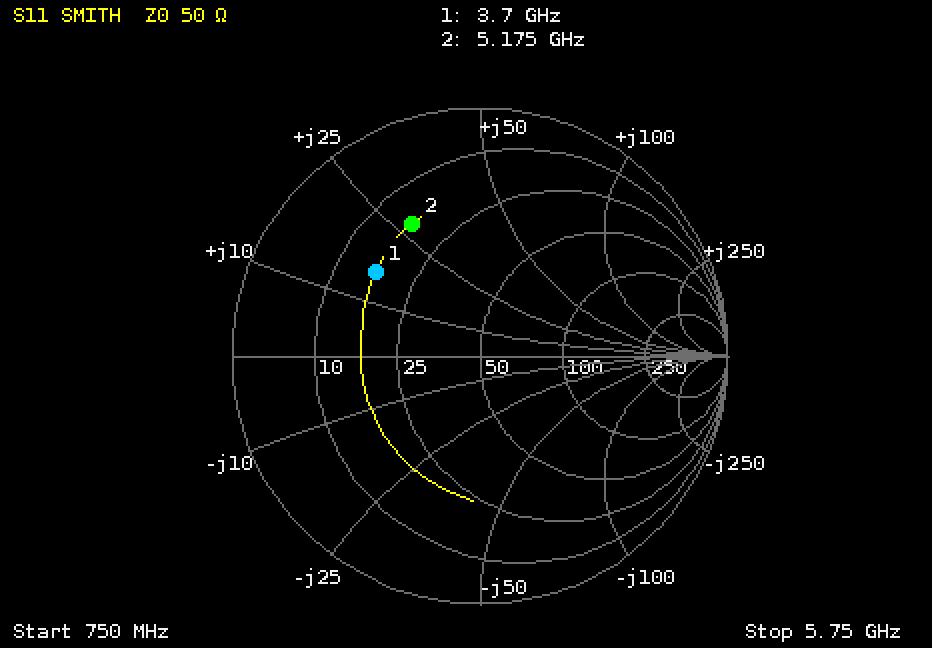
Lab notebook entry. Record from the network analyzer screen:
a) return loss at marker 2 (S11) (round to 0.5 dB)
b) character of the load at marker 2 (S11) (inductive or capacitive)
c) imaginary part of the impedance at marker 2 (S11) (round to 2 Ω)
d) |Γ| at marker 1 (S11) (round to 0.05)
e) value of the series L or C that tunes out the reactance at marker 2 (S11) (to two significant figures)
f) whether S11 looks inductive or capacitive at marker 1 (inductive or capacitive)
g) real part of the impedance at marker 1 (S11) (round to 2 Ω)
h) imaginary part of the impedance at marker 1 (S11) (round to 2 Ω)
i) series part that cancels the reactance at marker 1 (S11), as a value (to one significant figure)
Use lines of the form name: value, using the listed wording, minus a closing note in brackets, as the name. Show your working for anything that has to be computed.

return loss at marker 2 (S11): 4.5 dB
character of the load at marker 2 (S11): inductive
imaginary part of the impedance at marker 2 (S11): +28 Ω
|Γ| at marker 1 (S11): 0.55
value of the series L or C that tunes out the reactance at marker 2 (S11): C = 1/(2π × 5.175 GHz × 28 Ω) ≈ 1.1 pF
whether S11 looks inductive or capacitive at marker 1: inductive
real part of the impedance at marker 1 (S11): 16 Ω
imaginary part of the impedance at marker 1 (S11): +16 Ω
series part that cancels the reactance at marker 1 (S11), as a value: C = 1/(2π × 3.7 GHz × 16 Ω) ≈ 3 pF
